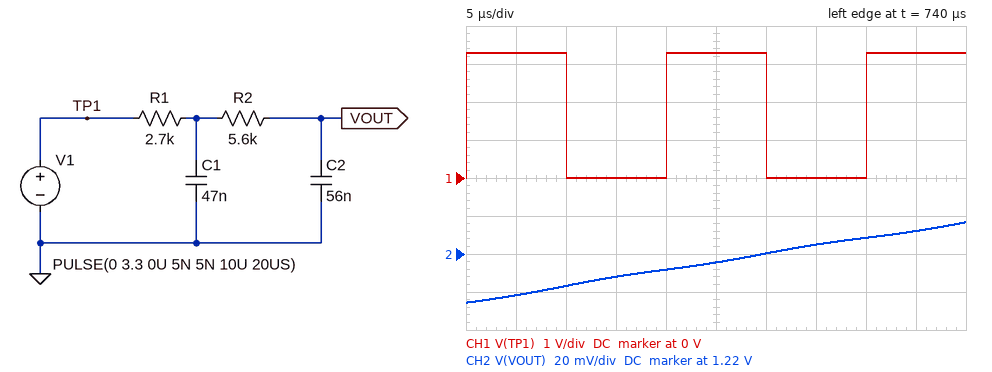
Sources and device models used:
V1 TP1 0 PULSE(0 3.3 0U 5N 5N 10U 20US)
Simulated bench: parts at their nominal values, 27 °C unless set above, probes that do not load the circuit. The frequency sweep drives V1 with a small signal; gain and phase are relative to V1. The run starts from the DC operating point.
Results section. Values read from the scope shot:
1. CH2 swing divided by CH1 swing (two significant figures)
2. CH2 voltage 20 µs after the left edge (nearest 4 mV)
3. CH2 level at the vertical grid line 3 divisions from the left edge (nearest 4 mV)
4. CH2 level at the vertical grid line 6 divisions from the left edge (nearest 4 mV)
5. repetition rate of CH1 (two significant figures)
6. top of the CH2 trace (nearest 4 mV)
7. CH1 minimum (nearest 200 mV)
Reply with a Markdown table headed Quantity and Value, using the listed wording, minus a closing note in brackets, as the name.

| Quantity | Value |
|---|---|
| CH2 swing divided by CH1 swing | 0.013 |
| CH2 voltage 20 µs after the left edge | 1.212 V |
| CH2 level at the vertical grid line 3 divisions from the left edge | 1.208 V |
| CH2 level at the vertical grid line 6 divisions from the left edge | 1.220 V |
| repetition rate of CH1 | 50 kHz |
| top of the CH2 trace | 1.236 V |
| CH1 minimum | 0 V |
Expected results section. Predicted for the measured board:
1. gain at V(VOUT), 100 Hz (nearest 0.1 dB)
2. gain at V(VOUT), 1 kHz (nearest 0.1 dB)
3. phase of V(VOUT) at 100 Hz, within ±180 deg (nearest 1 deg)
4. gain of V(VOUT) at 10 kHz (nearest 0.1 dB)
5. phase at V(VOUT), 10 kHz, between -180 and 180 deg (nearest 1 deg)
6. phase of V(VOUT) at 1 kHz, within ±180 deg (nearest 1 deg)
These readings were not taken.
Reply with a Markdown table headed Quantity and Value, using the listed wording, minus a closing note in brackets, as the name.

| Quantity | Value |
|---|---|
| gain at V(VOUT), 100 Hz | -0.4 dB |
| gain at V(VOUT), 1 kHz | -11.5 dB |
| phase of V(VOUT) at 100 Hz, within ±180 deg | -21 deg |
| gain of V(VOUT) at 10 kHz | -44.1 dB |
| phase at V(VOUT), 10 kHz, between -180 and 180 deg | -167 deg |
| phase of V(VOUT) at 1 kHz, within ±180 deg | -99 deg |
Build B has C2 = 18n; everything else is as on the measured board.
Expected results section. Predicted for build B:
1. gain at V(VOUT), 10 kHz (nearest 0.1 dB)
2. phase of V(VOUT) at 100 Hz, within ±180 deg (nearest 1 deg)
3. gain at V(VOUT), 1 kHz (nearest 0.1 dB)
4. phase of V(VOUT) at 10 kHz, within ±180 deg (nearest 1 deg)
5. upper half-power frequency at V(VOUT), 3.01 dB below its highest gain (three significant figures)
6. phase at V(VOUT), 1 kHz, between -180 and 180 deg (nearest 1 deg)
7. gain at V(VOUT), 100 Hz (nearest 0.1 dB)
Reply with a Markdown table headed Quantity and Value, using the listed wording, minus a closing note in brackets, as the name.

| Quantity | Value |
|---|---|
| gain at V(VOUT), 10 kHz | -34.4 dB |
| phase of V(VOUT) at 100 Hz, within ±180 deg | -10 deg |
| gain at V(VOUT), 1 kHz | -5.1 dB |
| phase of V(VOUT) at 10 kHz, within ±180 deg | -161 deg |
| upper half-power frequency at V(VOUT), 3.01 dB below its highest gain | 686 Hz |
| phase at V(VOUT), 1 kHz, between -180 and 180 deg | -74 deg |
| gain at V(VOUT), 100 Hz | -0.1 dB |
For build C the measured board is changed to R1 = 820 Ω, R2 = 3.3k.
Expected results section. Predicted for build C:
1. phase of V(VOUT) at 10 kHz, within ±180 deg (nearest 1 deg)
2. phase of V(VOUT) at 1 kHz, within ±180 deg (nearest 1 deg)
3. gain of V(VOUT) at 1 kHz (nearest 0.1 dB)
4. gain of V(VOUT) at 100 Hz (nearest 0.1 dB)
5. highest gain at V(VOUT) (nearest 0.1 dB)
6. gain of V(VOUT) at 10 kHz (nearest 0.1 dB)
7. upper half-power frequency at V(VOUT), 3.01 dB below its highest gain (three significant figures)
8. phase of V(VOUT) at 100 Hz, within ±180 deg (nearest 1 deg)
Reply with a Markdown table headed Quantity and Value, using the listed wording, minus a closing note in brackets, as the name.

| Quantity | Value |
|---|---|
| phase of V(VOUT) at 10 kHz, within ±180 deg | -148 deg |
| phase of V(VOUT) at 1 kHz, within ±180 deg | -67 deg |
| gain of V(VOUT) at 1 kHz | -5.3 dB |
| gain of V(VOUT) at 100 Hz | -0.1 dB |
| highest gain at V(VOUT) | 0 dB |
| gain of V(VOUT) at 10 kHz | -30.1 dB |
| upper half-power frequency at V(VOUT), 3.01 dB below its highest gain | 655 Hz |
| phase of V(VOUT) at 100 Hz, within ±180 deg | -10 deg |
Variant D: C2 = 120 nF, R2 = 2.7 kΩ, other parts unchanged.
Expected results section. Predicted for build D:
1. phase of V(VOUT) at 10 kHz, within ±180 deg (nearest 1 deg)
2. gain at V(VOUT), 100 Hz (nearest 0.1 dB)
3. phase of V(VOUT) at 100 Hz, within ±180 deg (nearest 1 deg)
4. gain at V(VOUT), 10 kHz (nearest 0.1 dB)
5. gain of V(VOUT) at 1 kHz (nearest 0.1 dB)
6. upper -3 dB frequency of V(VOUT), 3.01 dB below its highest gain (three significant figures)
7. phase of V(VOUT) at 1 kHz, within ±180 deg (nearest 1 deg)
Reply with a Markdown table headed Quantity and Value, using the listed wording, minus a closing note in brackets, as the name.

| Quantity | Value |
|---|---|
| phase of V(VOUT) at 10 kHz, within ±180 deg | -163 deg |
| gain at V(VOUT), 100 Hz | -0.8 dB |
| phase of V(VOUT) at 100 Hz, within ±180 deg | -26 deg |
| gain at V(VOUT), 10 kHz | -44.5 dB |
| gain of V(VOUT) at 1 kHz | -13.8 dB |
| upper -3 dB frequency of V(VOUT), 3.01 dB below its highest gain | 220 Hz |
| phase of V(VOUT) at 1 kHz, within ±180 deg | -97 deg |
